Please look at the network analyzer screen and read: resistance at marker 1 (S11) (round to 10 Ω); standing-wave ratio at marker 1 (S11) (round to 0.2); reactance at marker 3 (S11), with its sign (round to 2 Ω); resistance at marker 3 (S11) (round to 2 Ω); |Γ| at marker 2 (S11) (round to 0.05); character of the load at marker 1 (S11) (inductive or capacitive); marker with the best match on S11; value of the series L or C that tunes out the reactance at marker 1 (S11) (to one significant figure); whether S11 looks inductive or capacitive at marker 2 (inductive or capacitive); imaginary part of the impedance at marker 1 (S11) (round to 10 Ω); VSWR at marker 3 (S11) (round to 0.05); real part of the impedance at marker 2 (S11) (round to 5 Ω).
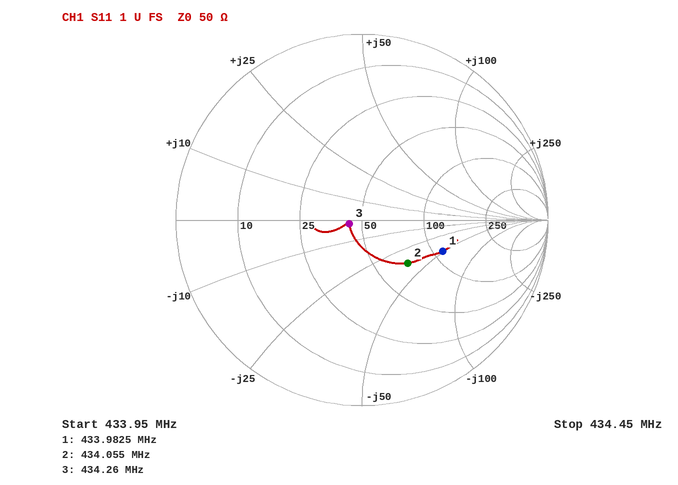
110 Ω
2.8
-2 Ω
44 Ω
0.35
capacitive
marker 3
20 nH
capacitive
-50 Ω
1.15
70 Ω
